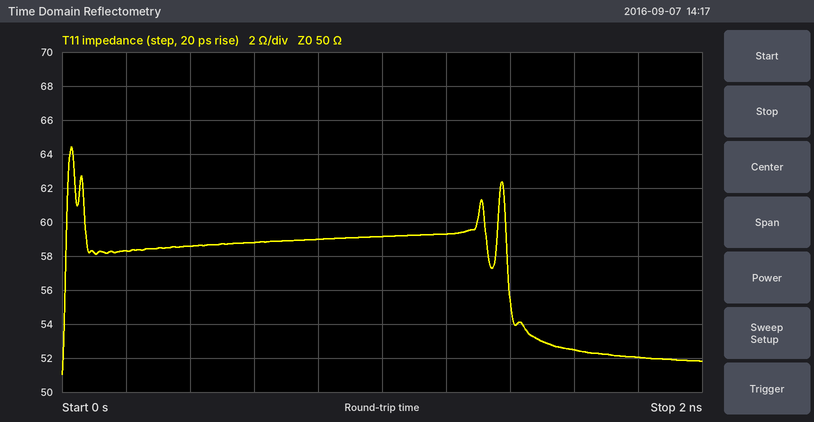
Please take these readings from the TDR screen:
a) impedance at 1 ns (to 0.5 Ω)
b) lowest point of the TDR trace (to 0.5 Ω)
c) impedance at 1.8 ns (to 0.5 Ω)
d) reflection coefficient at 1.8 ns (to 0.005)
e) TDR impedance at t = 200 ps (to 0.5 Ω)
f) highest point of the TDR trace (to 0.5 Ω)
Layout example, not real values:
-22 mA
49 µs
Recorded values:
59.0 Ω
51.0 Ω
52.0 Ω
+0.020
58.5 Ω
64.5 Ω
